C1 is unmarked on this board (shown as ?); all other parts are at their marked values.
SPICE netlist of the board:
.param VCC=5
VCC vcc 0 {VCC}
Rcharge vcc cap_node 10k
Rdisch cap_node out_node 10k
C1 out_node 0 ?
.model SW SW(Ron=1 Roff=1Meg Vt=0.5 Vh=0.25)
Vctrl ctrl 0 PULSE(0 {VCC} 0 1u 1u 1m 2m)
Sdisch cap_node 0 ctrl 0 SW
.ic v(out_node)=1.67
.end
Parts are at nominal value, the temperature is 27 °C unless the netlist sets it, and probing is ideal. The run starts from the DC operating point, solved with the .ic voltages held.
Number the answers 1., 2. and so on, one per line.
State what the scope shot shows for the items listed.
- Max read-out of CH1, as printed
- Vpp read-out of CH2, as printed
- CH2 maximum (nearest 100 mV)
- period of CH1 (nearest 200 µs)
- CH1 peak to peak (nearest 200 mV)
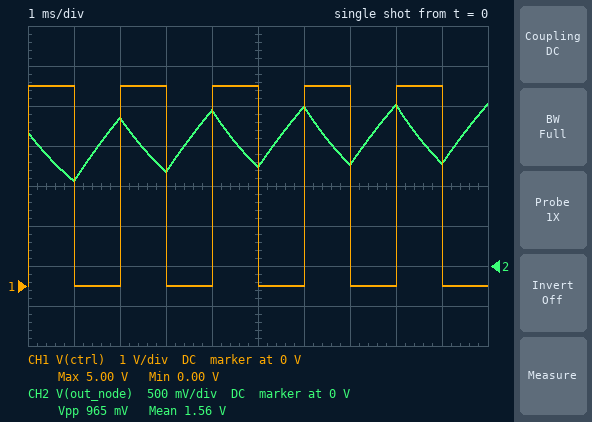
1. 5.00 V
2. 965 mV
3. 2.0 V
4. 2.0 ms
5. 5.0 V
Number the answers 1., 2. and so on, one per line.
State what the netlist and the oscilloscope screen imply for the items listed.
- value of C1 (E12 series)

1. 220 nF
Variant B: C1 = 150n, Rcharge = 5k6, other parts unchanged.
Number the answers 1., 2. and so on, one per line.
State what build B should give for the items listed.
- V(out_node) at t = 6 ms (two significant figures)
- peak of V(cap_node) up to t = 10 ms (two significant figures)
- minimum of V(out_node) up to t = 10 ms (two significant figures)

1. 2.6 V
2. 4.1 V
3. 860 mV
